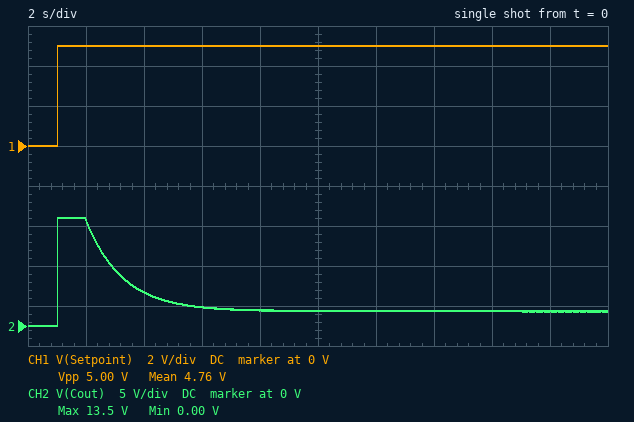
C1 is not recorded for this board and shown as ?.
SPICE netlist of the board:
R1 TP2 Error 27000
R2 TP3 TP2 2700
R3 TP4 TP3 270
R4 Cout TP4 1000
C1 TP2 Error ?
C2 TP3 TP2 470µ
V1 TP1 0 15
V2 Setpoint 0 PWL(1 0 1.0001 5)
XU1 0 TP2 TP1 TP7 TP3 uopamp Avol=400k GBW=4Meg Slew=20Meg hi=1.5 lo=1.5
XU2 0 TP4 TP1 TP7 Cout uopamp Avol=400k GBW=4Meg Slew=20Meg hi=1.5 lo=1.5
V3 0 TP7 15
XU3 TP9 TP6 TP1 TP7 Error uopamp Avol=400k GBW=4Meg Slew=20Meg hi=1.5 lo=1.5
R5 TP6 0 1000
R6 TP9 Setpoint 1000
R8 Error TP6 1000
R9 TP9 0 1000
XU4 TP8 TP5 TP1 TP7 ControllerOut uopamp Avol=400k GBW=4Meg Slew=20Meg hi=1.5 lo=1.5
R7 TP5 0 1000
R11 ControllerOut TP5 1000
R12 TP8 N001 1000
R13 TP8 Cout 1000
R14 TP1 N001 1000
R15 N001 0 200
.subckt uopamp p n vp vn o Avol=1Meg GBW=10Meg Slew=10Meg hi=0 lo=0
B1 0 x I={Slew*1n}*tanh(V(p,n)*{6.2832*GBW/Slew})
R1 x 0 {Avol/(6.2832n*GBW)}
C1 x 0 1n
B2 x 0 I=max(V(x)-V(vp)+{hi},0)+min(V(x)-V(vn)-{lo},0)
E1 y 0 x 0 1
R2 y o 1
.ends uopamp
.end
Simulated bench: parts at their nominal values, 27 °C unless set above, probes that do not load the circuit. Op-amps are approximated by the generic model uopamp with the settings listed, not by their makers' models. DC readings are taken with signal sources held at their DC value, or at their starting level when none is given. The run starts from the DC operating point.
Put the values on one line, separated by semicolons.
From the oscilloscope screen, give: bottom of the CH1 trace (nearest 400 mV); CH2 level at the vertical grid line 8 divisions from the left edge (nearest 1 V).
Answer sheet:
0 V; 2 V
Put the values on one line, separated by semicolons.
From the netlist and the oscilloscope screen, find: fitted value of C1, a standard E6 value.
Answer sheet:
680 µF
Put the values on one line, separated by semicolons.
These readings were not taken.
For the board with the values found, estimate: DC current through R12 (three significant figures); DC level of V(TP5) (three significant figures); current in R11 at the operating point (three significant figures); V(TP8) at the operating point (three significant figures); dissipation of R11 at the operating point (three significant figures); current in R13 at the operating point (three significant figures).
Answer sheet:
1.15 mA; 1.15 V; 1.15 mA; 1.15 V; 1.33 mW; 1.15 mA
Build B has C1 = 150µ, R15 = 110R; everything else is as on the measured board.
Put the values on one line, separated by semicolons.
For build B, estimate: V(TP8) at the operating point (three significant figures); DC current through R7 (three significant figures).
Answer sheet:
708 mV; 708 µA
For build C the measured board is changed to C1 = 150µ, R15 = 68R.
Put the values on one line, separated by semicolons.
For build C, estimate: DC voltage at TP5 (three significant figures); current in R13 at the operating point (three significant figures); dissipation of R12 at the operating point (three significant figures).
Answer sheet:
463 mV; 463 µA; 214 µW
